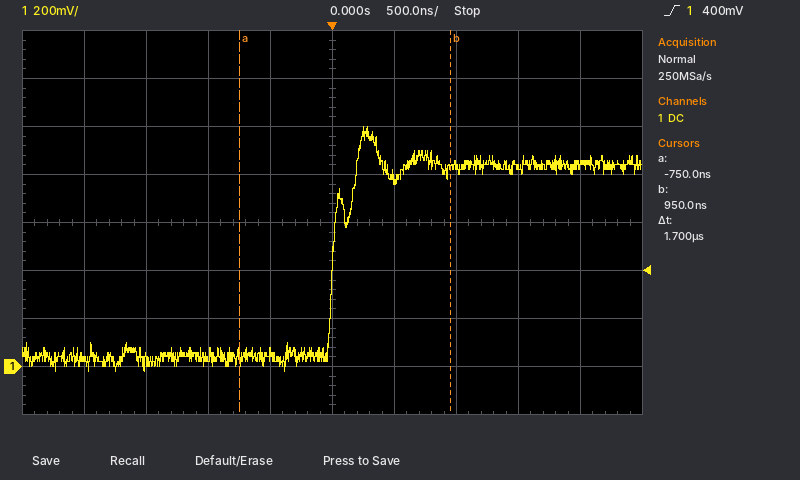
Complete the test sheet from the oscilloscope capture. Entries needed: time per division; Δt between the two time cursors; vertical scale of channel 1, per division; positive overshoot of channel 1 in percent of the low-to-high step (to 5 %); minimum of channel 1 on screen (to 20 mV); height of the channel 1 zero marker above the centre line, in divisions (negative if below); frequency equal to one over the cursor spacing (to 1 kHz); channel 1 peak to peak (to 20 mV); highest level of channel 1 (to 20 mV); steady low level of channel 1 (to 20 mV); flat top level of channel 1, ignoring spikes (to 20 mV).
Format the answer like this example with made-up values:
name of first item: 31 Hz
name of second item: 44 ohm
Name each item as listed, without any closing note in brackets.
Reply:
time per division: 500 ns
Δt between the two time cursors: 1.7 µs
vertical scale of channel 1, per division: 200 mV
positive overshoot of channel 1 in percent of the low-to-high step: 20 %
minimum of channel 1 on screen: -20 mV
height of the channel 1 zero marker above the centre line, in divisions: -3.0 div
frequency equal to one over the cursor spacing: 588 kHz
channel 1 peak to peak: 1.02 V
highest level of channel 1: 1.00 V
steady low level of channel 1: 40 mV
flat top level of channel 1, ignoring spikes: 840 mV
